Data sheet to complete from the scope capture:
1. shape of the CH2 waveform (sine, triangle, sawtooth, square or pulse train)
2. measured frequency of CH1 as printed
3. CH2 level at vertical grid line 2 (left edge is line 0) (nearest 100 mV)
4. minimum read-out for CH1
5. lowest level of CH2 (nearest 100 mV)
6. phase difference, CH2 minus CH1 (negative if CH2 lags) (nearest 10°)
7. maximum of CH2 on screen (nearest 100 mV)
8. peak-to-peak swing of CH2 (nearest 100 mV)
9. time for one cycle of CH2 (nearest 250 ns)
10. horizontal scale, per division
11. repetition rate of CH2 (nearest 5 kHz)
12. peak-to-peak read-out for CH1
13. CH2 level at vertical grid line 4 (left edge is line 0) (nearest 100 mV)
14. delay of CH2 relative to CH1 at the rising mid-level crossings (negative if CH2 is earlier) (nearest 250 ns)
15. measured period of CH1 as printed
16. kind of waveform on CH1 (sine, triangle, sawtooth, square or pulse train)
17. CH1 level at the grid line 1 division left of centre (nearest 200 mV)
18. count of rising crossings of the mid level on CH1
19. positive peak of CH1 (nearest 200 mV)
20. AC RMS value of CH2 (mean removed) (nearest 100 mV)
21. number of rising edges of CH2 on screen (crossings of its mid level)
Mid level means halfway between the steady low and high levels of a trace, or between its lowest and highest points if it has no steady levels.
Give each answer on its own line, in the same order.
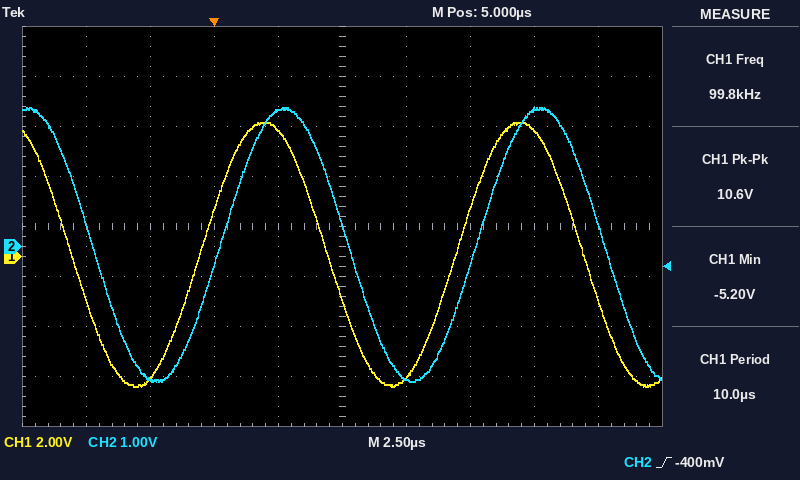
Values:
sine
99.8 kHz
-2.7 V
-5.20 V
-2.7 V
-30°
2.8 V
5.5 V
10.00 µs
2.5 µs
100 kHz
10.6 V
2.7 V
+750 ns
10.0 µs
sine
5.0 V
2
5.4 V
1.9 V
2
